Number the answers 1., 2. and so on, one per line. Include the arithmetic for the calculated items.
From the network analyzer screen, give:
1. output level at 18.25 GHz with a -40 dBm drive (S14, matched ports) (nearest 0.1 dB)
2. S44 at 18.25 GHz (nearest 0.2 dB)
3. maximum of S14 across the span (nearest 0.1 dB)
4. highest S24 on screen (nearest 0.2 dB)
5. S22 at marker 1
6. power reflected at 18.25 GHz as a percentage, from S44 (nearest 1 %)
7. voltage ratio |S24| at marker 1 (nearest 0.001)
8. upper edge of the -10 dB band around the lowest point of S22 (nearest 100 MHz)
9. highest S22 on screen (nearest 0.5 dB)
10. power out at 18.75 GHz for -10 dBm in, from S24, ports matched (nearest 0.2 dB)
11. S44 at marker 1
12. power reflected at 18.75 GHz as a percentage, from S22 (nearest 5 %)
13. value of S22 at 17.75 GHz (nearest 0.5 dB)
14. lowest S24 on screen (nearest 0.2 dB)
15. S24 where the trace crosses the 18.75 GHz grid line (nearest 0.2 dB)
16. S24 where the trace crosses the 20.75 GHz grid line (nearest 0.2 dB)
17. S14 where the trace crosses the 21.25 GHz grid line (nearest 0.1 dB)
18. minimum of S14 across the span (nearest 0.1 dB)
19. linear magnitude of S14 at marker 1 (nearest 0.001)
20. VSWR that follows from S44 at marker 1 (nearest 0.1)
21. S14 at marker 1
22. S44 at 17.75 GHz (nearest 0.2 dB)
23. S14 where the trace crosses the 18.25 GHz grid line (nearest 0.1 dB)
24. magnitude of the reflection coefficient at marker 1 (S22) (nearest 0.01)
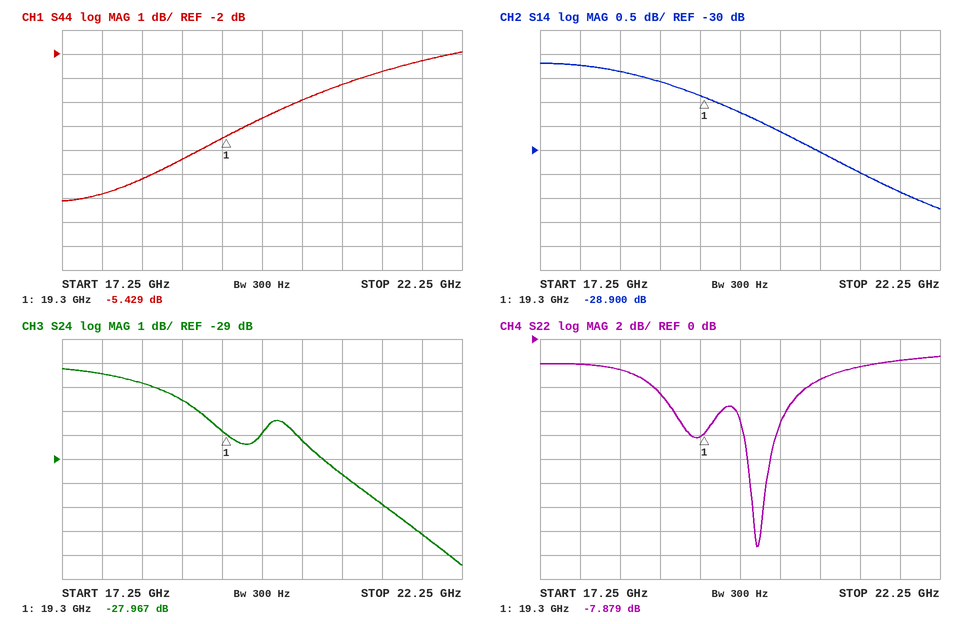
1. -40 dBm + (-28.4 dB) = -68.4 dBm
2. -7.2 dB
3. -28.2 dB
4. -25.2 dB
5. -7.879 dB
6. 10^(-7.2/10) ≈ 19 %
7. 10^(-27.967/20) ≈ 0.040
8. 20.1 GHz
9. -1.5 dB
10. -10 dBm + (-26.6 dB) = -36.6 dBm
11. -5.429 dB
12. 10^(-4.5/10) ≈ 35 %
13. -2.0 dB
14. -33.4 dB
15. -26.6 dB
16. -29.6 dB
17. -30.5 dB
18. -31.2 dB
19. 10^(-28.9/20) ≈ 0.036
20. (1 + 0.5352)/(1 − 0.5352) ≈ 3.3
21. -28.900 dB
22. -7.8 dB
23. -28.4 dB
24. 10^(-7.879/20) ≈ 0.40
